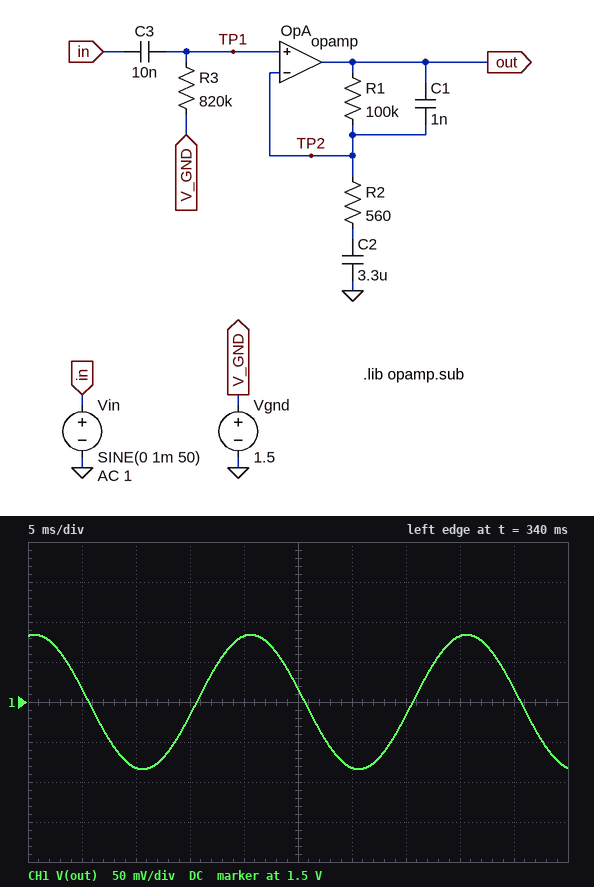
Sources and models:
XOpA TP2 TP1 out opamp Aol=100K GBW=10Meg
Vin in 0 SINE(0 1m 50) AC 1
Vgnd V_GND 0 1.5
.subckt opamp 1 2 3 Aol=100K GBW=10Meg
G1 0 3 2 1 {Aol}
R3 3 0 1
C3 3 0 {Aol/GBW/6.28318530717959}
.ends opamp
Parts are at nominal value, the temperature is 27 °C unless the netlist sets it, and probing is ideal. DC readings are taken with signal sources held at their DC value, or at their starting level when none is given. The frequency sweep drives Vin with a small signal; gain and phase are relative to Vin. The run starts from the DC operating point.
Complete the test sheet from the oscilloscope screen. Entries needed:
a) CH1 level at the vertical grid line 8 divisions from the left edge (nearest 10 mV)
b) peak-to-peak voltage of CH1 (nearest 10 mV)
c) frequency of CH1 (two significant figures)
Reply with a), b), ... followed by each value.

a) 1.58 V
b) 170 mV
c) 50 Hz
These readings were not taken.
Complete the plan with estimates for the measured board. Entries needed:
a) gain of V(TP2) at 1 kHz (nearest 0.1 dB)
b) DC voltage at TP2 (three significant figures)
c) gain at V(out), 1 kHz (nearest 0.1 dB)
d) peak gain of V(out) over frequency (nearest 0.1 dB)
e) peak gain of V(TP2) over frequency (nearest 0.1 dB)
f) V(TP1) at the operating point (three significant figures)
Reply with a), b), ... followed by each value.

a) -0.1 dB
b) 1.50 V
c) 43.5 dB
d) 44.6 dB
e) 0 dB
f) 1.50 V
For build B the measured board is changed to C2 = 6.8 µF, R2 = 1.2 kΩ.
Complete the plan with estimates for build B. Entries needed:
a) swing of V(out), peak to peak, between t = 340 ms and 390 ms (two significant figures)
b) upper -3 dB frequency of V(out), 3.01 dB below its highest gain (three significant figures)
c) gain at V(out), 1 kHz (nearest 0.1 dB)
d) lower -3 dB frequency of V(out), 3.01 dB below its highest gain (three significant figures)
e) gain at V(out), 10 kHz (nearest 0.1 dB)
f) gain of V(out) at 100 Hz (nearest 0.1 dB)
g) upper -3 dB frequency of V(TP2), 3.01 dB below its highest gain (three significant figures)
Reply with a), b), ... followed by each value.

a) 150 mV
b) 1.63 kHz
c) 37.0 dB
d) 29.4 Hz
e) 22.4 dB
f) 38.2 dB
g) 9.92 MHz
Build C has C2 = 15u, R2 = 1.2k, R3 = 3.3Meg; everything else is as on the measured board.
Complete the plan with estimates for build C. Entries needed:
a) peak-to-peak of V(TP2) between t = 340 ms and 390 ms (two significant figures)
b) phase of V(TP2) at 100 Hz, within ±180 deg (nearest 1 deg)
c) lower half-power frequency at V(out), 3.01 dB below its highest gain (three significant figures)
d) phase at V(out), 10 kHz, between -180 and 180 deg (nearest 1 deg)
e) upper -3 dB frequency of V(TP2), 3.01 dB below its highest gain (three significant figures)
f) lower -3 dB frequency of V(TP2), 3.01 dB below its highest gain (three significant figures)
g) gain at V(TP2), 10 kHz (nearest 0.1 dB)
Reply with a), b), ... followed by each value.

a) 2.0 mV
b) 3 deg
c) 10.7 Hz
d) -77 deg
e) 9.89 MHz
f) 4.81 Hz
g) -0.1 dB
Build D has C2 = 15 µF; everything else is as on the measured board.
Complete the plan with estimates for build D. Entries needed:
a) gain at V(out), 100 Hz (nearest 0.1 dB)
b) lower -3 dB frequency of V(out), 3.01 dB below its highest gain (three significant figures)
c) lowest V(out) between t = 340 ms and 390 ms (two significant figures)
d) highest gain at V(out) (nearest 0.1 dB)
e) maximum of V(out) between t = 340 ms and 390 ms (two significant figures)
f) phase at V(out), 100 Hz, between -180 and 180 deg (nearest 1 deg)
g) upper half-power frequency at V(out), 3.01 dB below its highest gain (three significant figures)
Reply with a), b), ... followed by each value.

a) 44.7 dB
b) 28.9 Hz
c) 1.3 V
d) 44.9 dB
e) 1.7 V
f) 18 deg
g) 1.60 kHz
